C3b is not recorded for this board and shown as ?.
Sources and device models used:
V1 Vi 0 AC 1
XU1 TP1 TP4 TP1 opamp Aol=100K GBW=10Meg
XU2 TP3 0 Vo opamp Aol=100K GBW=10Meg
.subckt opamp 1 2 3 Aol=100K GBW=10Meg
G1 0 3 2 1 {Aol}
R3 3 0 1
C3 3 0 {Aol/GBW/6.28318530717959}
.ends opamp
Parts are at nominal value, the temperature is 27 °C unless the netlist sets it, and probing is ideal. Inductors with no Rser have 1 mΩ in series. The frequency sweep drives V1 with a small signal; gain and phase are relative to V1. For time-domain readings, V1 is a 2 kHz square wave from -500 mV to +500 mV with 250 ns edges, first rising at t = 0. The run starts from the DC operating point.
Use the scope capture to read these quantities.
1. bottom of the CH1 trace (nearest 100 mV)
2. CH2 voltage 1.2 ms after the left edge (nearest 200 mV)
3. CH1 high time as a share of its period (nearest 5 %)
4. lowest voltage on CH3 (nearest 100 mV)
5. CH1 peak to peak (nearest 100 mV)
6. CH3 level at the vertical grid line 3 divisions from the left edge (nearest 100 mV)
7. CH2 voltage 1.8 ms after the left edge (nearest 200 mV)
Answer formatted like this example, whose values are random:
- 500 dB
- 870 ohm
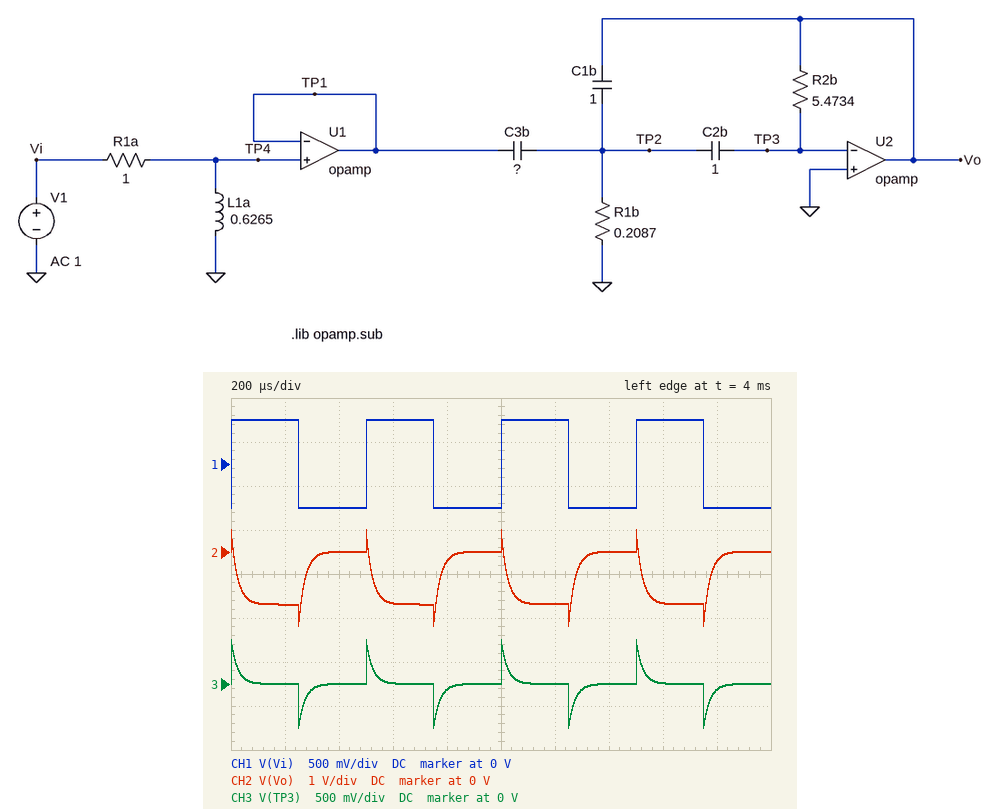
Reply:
- -500 mV
- -1.2 V
- 50 %
- -500 mV
- 1.0 V
- 0 V
- -200 mV
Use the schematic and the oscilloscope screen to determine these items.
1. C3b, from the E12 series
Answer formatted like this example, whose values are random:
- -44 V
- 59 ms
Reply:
- 1.2 F
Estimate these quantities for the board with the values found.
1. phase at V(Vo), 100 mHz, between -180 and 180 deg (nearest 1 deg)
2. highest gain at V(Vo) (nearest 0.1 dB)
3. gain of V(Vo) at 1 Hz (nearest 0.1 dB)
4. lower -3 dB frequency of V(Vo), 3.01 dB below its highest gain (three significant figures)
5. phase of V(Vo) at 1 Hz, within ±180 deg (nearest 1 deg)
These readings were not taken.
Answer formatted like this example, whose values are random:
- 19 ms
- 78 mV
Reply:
- 31 deg
- 1.6 dB
- 1.5 dB
- 140 mHz
- -160 deg
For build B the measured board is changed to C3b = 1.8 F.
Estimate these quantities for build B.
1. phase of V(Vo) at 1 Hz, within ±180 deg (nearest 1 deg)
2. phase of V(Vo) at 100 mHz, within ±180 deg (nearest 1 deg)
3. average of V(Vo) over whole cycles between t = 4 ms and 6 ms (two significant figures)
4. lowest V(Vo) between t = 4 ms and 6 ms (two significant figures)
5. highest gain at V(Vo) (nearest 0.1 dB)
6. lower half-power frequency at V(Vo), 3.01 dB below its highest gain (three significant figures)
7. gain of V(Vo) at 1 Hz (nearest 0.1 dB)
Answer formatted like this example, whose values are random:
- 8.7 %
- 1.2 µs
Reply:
- -159 deg
- 26 deg
- -890 mV
- -2.3 V
- 5.1 dB
- 152 mHz
- 5.0 dB
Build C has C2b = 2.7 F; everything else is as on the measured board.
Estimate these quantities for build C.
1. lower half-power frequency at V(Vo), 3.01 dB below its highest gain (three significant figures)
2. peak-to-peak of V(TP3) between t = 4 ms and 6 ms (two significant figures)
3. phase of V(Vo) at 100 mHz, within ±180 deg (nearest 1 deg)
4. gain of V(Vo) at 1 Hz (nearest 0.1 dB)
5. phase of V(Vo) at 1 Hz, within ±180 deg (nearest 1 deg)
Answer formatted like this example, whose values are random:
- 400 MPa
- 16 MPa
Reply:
- 163 mHz
- 990 mV
- -40 deg
- 1.4 dB
- -163 deg
